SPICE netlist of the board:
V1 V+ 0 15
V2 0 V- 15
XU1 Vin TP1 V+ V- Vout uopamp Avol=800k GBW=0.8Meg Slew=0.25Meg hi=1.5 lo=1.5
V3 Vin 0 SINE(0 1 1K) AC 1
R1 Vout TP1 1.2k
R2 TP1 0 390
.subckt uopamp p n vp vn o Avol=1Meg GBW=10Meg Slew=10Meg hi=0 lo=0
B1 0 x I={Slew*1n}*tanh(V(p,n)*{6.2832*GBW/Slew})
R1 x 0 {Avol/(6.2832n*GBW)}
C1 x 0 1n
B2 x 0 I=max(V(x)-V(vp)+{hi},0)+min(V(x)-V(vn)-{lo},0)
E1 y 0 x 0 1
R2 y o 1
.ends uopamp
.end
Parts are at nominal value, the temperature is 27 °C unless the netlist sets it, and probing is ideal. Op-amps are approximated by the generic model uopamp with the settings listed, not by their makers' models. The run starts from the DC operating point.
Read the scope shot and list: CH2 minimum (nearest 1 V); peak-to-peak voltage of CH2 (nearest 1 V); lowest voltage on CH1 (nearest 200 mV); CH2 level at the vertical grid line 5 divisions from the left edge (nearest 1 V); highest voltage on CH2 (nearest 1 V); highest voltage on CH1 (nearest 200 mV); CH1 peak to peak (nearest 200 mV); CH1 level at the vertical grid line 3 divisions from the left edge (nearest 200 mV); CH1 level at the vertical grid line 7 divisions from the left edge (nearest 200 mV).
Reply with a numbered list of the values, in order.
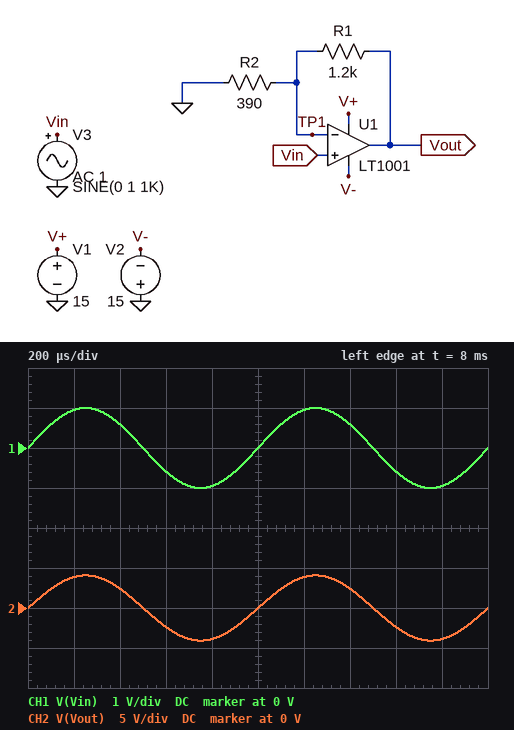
1. -4 V
2. 8 V
3. -1.0 V
4. 0 V
5. 4 V
6. 1.0 V
7. 2.0 V
8. -600 mV
9. 600 mV
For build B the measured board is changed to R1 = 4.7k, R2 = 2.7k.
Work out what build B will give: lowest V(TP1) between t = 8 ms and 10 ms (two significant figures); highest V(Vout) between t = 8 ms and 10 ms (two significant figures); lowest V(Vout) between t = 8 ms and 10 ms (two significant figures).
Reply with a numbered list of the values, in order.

1. -1.0 V
2. 2.7 V
3. -2.7 V
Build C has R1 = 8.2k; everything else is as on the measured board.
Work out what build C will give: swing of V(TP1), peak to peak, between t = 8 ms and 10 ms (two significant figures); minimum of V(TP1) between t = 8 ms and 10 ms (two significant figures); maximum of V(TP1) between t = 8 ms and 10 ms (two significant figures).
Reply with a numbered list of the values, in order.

1. 1.2 V
2. -610 mV
3. 610 mV
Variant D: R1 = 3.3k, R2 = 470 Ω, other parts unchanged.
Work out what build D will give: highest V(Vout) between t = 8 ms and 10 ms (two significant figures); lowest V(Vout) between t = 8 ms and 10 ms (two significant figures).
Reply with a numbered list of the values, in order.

1. 8.0 V
2. -8.0 V
